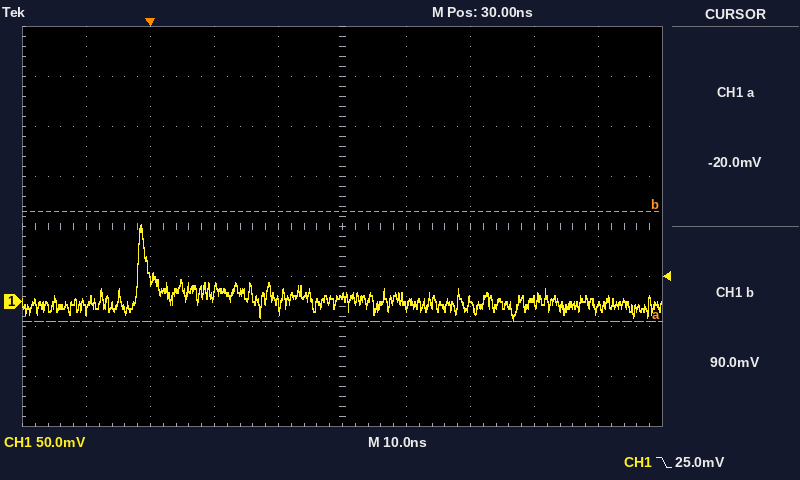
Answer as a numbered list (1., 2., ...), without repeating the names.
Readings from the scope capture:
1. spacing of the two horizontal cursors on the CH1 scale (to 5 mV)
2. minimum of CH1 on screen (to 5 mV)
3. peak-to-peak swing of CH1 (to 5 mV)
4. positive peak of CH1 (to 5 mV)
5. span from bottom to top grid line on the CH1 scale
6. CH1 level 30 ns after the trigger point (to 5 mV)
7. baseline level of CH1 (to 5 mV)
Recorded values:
1. 110 mV
2. -20 mV
3. 95 mV
4. 75 mV
5. 400 mV
6. 5 mV
7. 0 mV
